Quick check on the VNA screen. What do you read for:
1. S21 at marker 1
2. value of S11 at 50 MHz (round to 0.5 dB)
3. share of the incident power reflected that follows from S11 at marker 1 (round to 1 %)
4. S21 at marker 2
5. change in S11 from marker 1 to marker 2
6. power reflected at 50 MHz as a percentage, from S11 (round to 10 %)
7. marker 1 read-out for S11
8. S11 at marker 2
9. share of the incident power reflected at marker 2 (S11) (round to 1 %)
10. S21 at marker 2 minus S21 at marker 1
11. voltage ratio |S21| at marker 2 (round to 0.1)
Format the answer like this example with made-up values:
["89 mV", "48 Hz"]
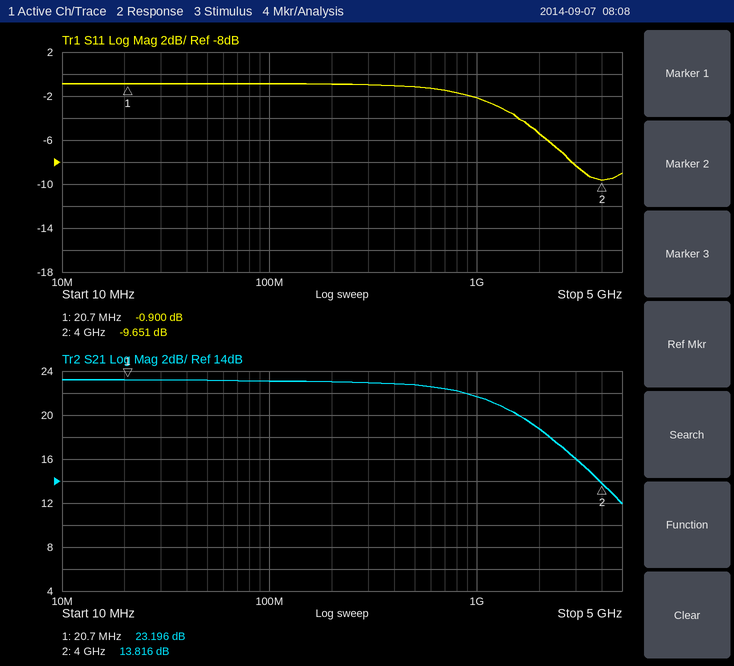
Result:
["23.196 dB", "-1.0 dB", "81 %", "13.816 dB", "-8.751 dB", "80 %", "-0.900 dB", "-9.651 dB", "11 %", "-9.380 dB", "4.9"]
